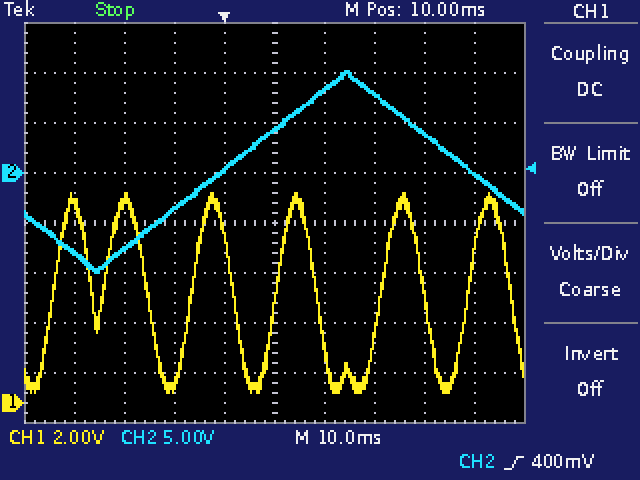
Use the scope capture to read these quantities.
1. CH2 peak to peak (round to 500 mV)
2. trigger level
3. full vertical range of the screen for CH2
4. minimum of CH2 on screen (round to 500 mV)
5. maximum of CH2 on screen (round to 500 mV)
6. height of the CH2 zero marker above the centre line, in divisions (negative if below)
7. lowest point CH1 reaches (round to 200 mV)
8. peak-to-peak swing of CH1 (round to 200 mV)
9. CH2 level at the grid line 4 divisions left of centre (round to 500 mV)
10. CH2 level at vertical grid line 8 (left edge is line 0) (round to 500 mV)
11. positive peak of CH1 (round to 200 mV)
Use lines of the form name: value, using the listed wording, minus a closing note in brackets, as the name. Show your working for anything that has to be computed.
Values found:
CH2 peak to peak: 10.0 V − (-10.0 V) = 20.0 V
trigger level: 400 mV
full vertical range of the screen for CH2: 40 V
minimum of CH2 on screen: -10.0 V
maximum of CH2 on screen: 10.0 V
height of the CH2 zero marker above the centre line, in divisions: +1.0 div
lowest point CH1 reaches: 400 mV
peak-to-peak swing of CH1: 8.4 V − (400 mV) = 8.0 V
CH2 level at the grid line 4 divisions left of centre: -8.0 V
CH2 level at vertical grid line 8 (left edge is line 0): 4.0 V
positive peak of CH1: 8.4 V
